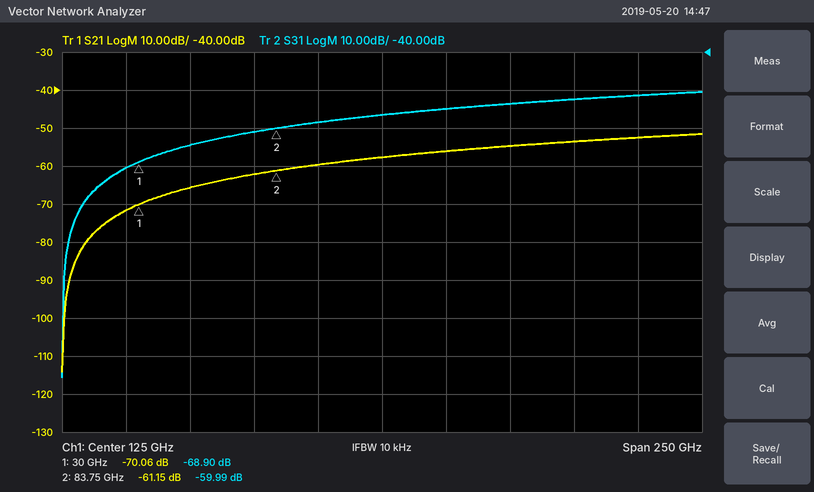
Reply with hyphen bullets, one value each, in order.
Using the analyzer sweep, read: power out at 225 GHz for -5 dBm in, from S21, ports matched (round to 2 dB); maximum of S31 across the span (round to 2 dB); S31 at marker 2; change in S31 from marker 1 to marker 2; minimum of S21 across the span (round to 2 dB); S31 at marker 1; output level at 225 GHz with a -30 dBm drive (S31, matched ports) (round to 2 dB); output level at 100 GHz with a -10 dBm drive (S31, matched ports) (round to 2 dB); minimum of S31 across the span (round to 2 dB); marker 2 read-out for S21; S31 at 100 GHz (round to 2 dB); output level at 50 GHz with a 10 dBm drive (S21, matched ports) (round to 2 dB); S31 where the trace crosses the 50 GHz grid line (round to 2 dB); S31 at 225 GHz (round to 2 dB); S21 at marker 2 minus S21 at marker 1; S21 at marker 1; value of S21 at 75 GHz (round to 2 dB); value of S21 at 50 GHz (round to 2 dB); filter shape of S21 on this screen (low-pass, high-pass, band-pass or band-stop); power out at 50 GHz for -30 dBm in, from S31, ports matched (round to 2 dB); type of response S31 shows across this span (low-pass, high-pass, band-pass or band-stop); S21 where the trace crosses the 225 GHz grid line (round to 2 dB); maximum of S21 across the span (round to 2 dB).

- -58 dBm
- -50 dB
- -59.99 dB
- 8.91 dB
- -114 dB
- -68.90 dB
- -82 dBm
- -68 dBm
- -126 dB
- -61.15 dB
- -58 dB
- -56 dBm
- -64 dB
- -52 dB
- 8.91 dB
- -70.06 dB
- -62 dB
- -66 dB
- high-pass
- -94 dBm
- high-pass
- -52 dB
- -52 dB
